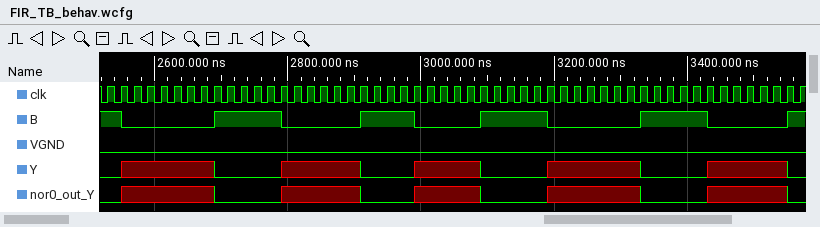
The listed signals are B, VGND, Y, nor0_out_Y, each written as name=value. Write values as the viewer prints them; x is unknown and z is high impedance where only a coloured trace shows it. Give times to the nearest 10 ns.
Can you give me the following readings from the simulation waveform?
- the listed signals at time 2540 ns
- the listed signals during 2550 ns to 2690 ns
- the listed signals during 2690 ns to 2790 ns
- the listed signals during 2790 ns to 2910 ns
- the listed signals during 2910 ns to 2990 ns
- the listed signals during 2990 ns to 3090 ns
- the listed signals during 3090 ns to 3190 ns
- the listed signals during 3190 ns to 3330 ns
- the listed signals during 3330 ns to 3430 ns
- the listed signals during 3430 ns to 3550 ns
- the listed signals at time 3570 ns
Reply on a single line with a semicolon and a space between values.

B=1, VGND=0, Y=0, nor0_out_Y=0; B=0, VGND=0, Y=x, nor0_out_Y=x; B=1, VGND=0, Y=0, nor0_out_Y=0; B=0, VGND=0, Y=x, nor0_out_Y=x; B=1, VGND=0, Y=0, nor0_out_Y=0; B=0, VGND=0, Y=x, nor0_out_Y=x; B=1, VGND=0, Y=0, nor0_out_Y=0; B=0, VGND=0, Y=x, nor0_out_Y=x; B=1, VGND=0, Y=0, nor0_out_Y=0; B=0, VGND=0, Y=x, nor0_out_Y=x; B=1, VGND=0, Y=0, nor0_out_Y=0
